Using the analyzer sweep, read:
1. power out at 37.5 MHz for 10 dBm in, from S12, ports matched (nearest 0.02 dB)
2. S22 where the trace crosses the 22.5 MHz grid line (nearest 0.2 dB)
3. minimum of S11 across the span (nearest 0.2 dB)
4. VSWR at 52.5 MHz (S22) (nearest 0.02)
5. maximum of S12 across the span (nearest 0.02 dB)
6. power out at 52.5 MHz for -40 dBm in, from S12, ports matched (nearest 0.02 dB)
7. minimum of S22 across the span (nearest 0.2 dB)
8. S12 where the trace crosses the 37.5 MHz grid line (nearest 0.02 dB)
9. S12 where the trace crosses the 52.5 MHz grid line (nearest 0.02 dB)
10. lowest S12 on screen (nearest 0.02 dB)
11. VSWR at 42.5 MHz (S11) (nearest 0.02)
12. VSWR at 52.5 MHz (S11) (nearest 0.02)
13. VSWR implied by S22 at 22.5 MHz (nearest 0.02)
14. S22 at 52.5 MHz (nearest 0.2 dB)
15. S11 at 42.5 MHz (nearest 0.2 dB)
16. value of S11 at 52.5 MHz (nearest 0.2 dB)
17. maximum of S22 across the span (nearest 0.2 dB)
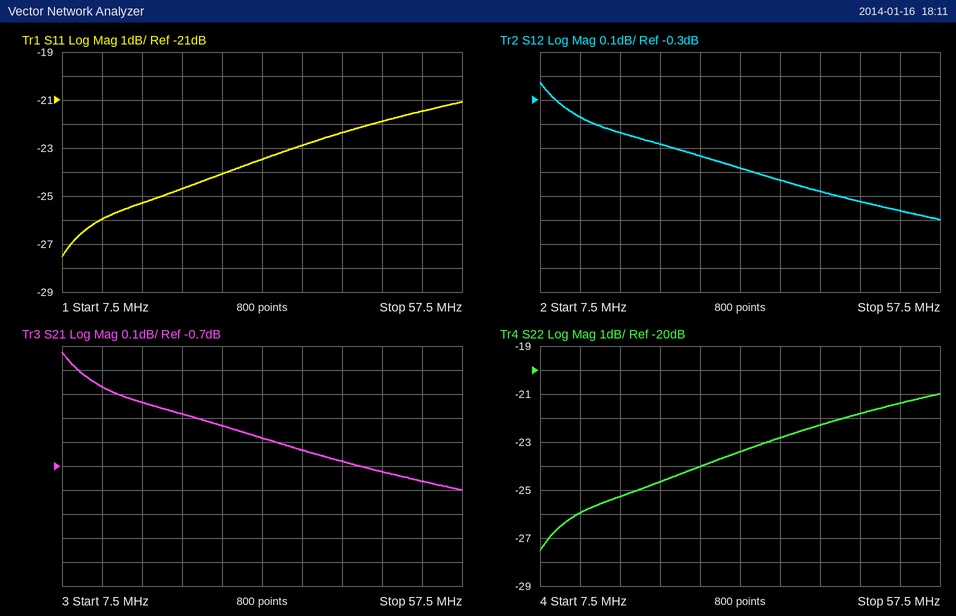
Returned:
9.36 dBm
-24.6 dB
-27.6 dB
1.18
-0.22 dB
-40.76 dBm
-27.6 dB
-0.64 dB
-0.76 dB
-0.80 dB
1.16
1.18
1.12
-21.4 dB
-22.4 dB
-21.4 dB
-21.0 dB
